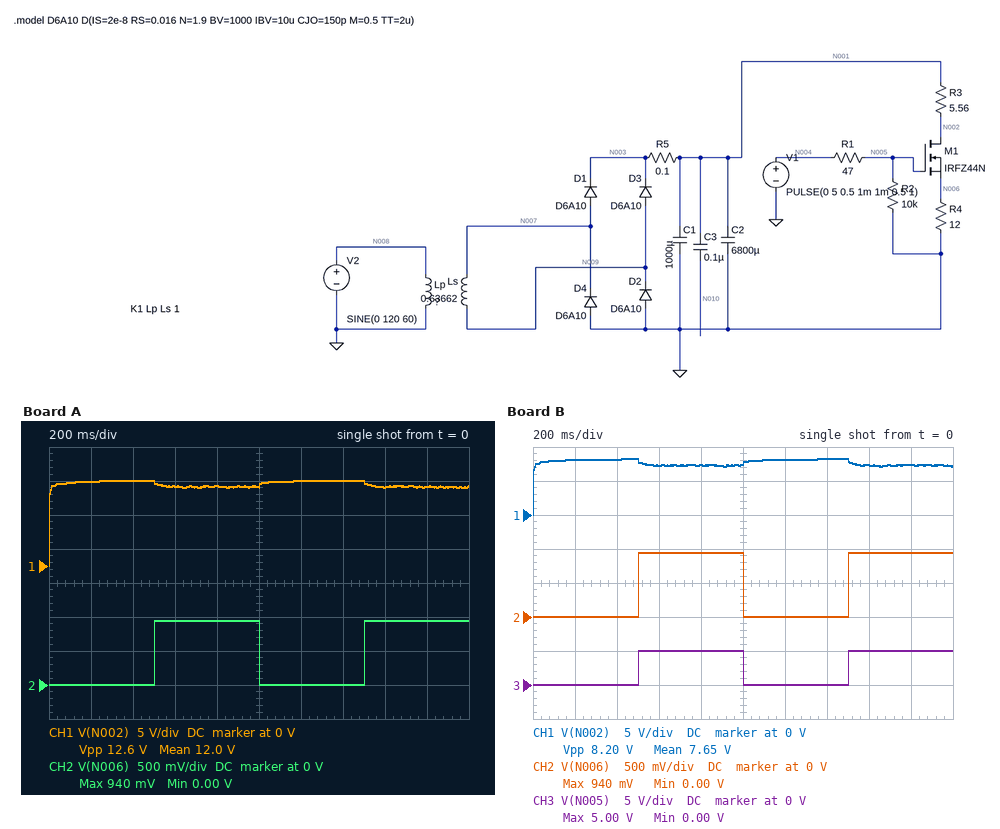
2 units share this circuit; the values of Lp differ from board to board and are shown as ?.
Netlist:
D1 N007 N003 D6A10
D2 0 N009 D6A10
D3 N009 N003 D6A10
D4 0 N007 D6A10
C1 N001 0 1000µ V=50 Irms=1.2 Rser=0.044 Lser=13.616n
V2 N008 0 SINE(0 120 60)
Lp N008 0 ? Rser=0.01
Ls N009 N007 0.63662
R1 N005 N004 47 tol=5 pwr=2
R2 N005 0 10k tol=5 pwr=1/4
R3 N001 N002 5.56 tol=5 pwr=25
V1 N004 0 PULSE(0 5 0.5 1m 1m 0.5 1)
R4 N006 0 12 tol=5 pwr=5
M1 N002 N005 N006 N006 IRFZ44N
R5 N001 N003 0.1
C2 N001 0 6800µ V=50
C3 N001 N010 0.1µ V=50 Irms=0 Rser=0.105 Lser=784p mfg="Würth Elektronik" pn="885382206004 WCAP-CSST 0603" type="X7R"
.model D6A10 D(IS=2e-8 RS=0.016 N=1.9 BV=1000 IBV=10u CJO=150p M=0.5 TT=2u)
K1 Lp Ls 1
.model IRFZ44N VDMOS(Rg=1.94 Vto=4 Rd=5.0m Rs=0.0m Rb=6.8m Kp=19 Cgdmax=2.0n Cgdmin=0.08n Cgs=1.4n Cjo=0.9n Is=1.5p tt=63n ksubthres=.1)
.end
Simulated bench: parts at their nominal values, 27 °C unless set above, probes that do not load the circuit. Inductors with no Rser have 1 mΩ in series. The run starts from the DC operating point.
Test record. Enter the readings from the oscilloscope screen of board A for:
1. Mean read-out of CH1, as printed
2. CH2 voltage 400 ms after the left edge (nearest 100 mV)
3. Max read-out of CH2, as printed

12.0 V
0 V
940 mV
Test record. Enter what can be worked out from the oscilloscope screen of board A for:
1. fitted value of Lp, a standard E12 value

47 H
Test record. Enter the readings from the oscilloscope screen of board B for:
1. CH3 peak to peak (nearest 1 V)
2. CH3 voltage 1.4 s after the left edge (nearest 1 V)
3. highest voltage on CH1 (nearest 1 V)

5 V
0 V
8 V
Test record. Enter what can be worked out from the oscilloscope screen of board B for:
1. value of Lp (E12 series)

100 H
